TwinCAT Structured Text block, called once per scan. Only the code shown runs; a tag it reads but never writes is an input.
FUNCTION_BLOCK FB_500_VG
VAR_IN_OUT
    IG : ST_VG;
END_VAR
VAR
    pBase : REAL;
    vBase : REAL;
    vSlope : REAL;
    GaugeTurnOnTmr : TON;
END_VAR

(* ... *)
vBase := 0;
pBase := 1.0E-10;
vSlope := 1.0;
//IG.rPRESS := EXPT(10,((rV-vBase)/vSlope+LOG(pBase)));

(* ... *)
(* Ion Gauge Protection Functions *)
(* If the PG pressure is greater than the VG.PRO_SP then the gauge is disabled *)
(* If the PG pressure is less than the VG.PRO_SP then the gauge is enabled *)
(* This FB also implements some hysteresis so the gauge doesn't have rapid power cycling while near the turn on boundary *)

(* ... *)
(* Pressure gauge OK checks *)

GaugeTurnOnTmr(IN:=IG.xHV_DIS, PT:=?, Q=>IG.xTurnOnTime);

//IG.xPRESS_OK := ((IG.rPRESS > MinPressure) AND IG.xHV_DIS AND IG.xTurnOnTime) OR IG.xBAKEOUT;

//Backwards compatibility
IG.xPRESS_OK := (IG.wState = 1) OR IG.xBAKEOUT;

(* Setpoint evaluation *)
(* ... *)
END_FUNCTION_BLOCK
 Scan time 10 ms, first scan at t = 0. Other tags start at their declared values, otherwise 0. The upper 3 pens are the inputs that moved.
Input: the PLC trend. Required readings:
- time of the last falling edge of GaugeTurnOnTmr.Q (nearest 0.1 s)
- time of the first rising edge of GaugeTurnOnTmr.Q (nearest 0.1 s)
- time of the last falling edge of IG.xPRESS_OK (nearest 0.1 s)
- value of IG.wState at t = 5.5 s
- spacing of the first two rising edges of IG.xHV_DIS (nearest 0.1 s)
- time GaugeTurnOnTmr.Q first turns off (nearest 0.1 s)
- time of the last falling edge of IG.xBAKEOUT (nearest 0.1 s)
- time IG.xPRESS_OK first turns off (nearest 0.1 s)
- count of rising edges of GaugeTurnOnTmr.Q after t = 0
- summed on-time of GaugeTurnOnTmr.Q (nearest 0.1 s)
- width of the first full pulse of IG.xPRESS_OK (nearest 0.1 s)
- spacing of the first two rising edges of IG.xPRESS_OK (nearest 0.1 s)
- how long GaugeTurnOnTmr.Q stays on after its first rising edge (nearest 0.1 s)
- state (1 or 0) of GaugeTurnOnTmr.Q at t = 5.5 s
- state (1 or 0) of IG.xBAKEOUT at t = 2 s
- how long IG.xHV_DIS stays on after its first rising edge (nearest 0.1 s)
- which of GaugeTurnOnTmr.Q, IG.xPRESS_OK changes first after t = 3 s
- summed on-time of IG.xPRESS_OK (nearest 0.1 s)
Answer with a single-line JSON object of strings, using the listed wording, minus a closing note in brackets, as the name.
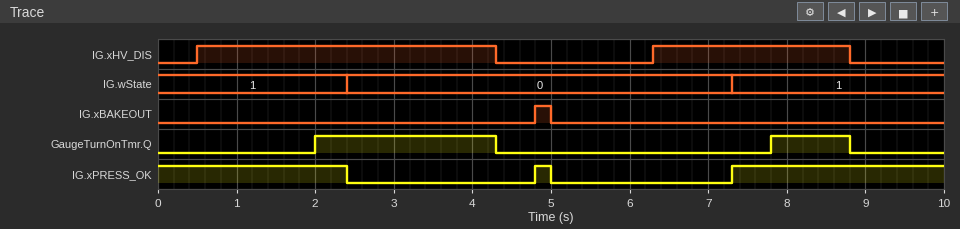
{"time of the last falling edge of GaugeTurnOnTmr.Q": "8.8 s", "time of the first rising edge of GaugeTurnOnTmr.Q": "2.0 s", "time of the last falling edge of IG.xPRESS_OK": "5.0 s", "value of IG.wState at t = 5.5 s": "0", "spacing of the first two rising edges of IG.xHV_DIS": "5.8 s", "time GaugeTurnOnTmr.Q first turns off": "4.3 s", "time of the last falling edge of IG.xBAKEOUT": "5.0 s", "time IG.xPRESS_OK first turns off": "2.4 s", "count of rising edges of GaugeTurnOnTmr.Q after t = 0": "2", "summed on-time of GaugeTurnOnTmr.Q": "3.3 s", "width of the first full pulse of IG.xPRESS_OK": "0.2 s", "spacing of the first two rising edges of IG.xPRESS_OK": "2.5 s", "how long GaugeTurnOnTmr.Q stays on after its first rising edge": "2.3 s", "state (1 or 0) of GaugeTurnOnTmr.Q at t = 5.5 s": "0", "state (1 or 0) of IG.xBAKEOUT at t = 2 s": "0", "how long IG.xHV_DIS stays on after its first rising edge": "3.8 s", "which of GaugeTurnOnTmr.Q, IG.xPRESS_OK changes first after t = 3 s": "GaugeTurnOnTmr.Q", "summed on-time of IG.xPRESS_OK": "5.3 s"}
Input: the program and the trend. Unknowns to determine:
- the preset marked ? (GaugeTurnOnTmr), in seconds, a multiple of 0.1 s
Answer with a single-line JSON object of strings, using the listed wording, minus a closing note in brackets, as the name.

{"the preset marked ? (GaugeTurnOnTmr), in seconds, a multiple of 0.1 s": "1.5 s"}
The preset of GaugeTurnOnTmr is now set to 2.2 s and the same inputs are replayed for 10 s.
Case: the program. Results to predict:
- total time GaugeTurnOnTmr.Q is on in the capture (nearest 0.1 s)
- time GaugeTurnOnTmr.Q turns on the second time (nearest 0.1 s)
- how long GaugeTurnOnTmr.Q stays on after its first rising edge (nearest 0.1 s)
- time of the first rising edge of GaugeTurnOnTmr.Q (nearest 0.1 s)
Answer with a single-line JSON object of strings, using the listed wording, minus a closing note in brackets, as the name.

{"total time GaugeTurnOnTmr.Q is on in the capture": "1.9 s", "time GaugeTurnOnTmr.Q turns on the second time": "8.5 s", "how long GaugeTurnOnTmr.Q stays on after its first rising edge": "1.6 s", "time of the first rising edge of GaugeTurnOnTmr.Q": "2.7 s"}
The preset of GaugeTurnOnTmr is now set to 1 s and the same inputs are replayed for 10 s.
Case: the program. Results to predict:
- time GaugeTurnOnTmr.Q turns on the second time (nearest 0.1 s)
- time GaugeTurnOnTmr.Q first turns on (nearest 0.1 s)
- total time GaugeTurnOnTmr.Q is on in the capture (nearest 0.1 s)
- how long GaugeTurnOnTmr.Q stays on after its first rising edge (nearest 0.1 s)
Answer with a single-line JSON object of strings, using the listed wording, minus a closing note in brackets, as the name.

{"time GaugeTurnOnTmr.Q turns on the second time": "7.3 s", "time GaugeTurnOnTmr.Q first turns on": "1.5 s", "total time GaugeTurnOnTmr.Q is on in the capture": "4.3 s", "how long GaugeTurnOnTmr.Q stays on after its first rising edge": "2.8 s"}
